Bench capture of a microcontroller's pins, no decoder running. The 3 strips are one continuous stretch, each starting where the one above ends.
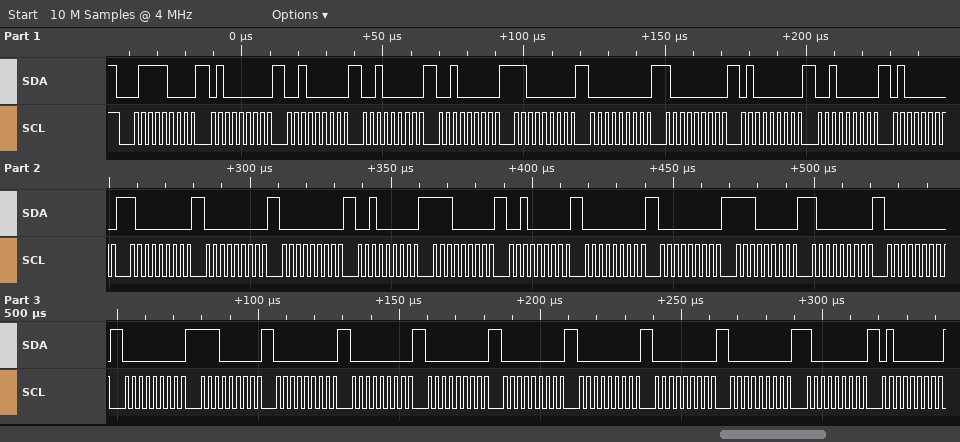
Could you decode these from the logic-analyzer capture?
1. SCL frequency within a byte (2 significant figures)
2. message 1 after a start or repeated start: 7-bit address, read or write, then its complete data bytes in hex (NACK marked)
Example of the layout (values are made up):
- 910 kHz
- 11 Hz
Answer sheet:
- 400 kHz
- 0x3C write: 40 20 20 20 C0 00 80 40 20 40 80 00 00 20 E0 20 00 00 E0 80 00 00 E0 00 00 00 00 00 00 00 80 40
